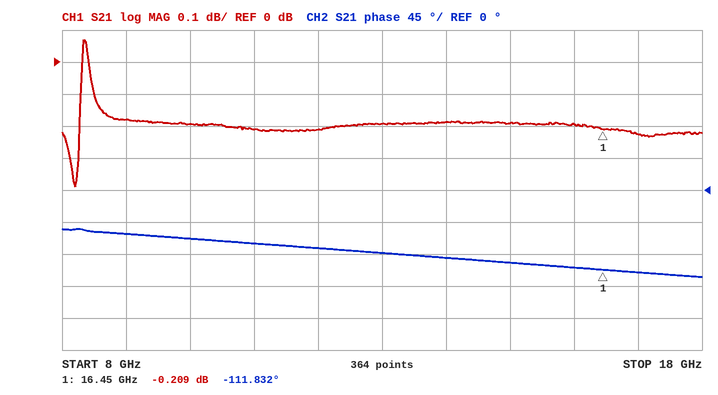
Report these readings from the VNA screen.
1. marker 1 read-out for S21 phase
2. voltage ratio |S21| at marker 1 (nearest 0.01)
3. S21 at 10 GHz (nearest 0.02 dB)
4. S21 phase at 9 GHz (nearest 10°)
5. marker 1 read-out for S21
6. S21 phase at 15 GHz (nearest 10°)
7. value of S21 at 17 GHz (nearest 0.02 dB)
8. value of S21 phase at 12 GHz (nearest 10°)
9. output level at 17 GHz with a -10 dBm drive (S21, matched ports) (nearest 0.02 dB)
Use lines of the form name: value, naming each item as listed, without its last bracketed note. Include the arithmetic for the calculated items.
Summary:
marker 1 read-out for S21 phase: -111.832°
voltage ratio |S21| at marker 1: 10^(-0.209/20) ≈ 0.98
S21 at 10 GHz: -0.20 dB
S21 phase at 9 GHz: -60°
marker 1 read-out for S21: -0.209 dB
S21 phase at 15 GHz: -100°
value of S21 at 17 GHz: -0.22 dB
value of S21 phase at 12 GHz: -80°
output level at 17 GHz with a -10 dBm drive (S21, matched ports): -10 dBm + (-0.22 dB) = -10.22 dBm
